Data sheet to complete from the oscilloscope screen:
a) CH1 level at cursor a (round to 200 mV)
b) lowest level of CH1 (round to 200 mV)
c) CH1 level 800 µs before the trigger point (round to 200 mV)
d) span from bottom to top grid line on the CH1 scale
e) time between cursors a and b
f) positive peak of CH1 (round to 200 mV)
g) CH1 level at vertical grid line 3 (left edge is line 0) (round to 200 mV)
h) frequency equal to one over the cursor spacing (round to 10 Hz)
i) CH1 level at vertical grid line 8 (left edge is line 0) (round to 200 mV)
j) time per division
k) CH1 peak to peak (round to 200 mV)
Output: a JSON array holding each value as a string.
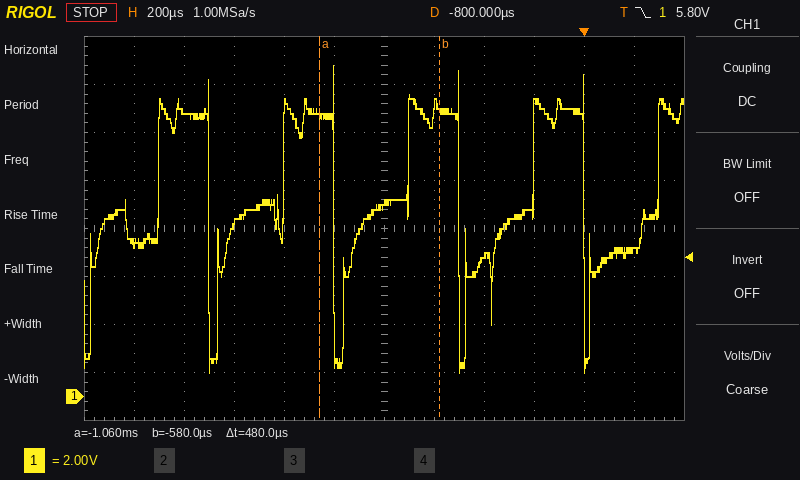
["11.8 V", "1.0 V", "8.0 V", "16 V", "480 µs", "13.8 V", "7.2 V", "2.08 kHz", "5.8 V", "200 µs", "12.8 V"]
